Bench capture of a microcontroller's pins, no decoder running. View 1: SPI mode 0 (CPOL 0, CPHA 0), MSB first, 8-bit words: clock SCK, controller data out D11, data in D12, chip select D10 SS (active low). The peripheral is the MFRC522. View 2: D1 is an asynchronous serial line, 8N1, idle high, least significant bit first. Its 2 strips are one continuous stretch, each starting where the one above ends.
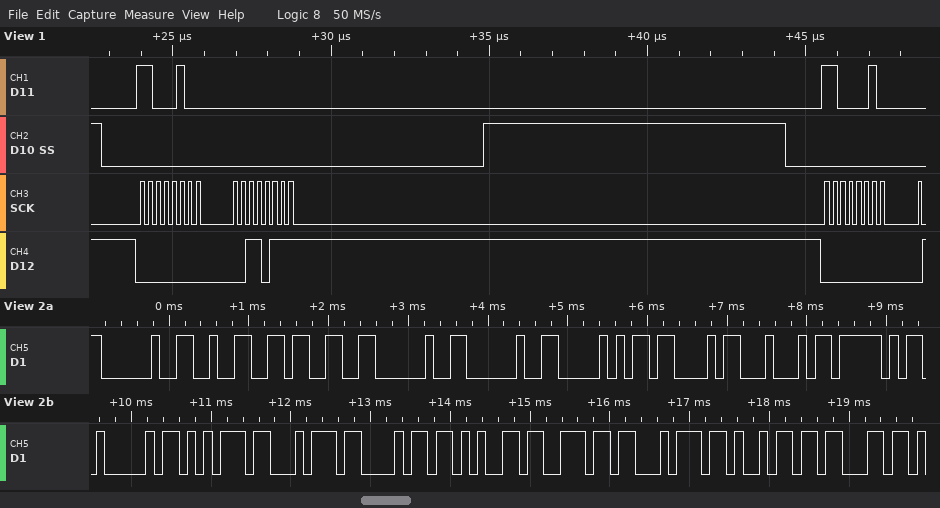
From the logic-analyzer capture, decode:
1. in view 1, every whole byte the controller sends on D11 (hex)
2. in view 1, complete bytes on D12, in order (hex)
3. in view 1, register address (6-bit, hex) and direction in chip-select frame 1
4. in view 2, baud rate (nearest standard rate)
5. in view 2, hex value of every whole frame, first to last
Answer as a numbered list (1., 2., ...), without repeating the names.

1. 0xC4 0x00 0xC2
2. 0x00 0x37 0x00
3. 0x22 read
4. 9600 baud
5. 20 32 33 20 20 50 43 44 5F 41 75 74 68 65 6E 74 69 63
